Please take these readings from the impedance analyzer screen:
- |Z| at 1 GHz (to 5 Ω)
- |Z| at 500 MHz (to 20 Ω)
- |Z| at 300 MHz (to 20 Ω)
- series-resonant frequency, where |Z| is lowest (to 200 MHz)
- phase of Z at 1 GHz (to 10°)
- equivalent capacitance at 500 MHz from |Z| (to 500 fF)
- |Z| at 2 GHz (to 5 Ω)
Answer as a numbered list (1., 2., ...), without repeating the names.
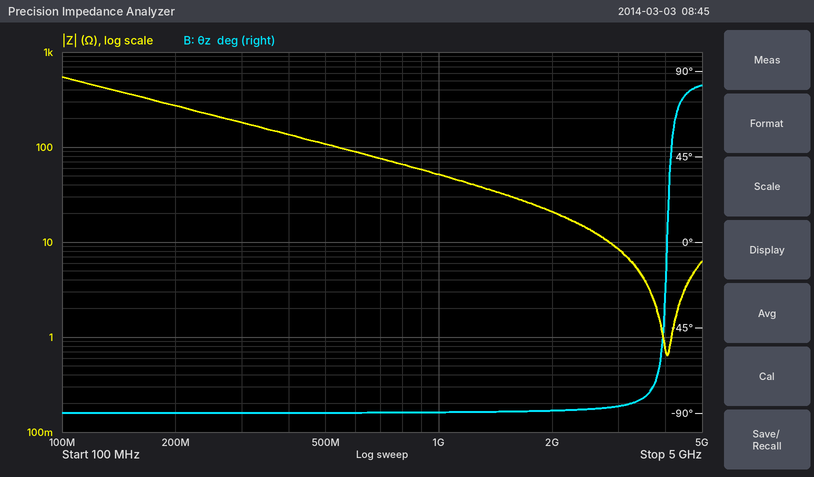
1. 50 Ω
2. 100 Ω
3. 180 Ω
4. 4.0 GHz
5. -90°
6. 3.0 pF
7. 20 Ω
